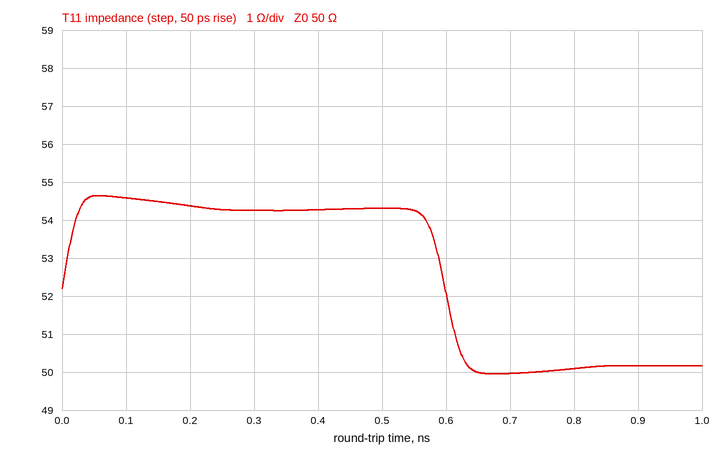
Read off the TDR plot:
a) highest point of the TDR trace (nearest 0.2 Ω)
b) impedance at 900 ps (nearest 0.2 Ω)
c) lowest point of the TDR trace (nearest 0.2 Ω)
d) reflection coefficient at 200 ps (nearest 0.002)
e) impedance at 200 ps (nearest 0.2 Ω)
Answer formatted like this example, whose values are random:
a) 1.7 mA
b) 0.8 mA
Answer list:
a) 54.6 Ω
b) 50.2 Ω
c) 50.0 Ω
d) +0.042
e) 54.4 Ω
